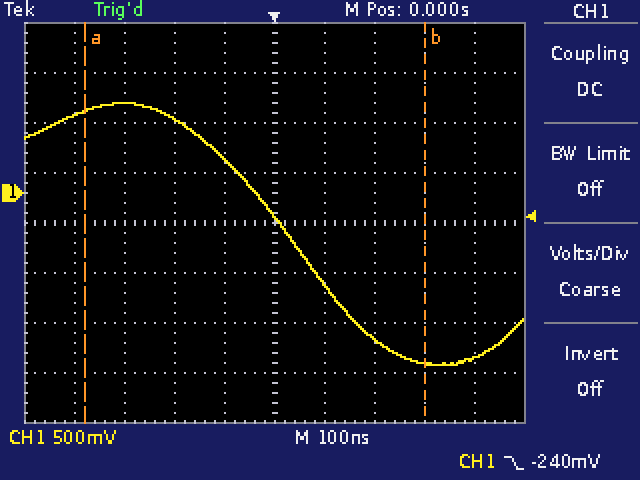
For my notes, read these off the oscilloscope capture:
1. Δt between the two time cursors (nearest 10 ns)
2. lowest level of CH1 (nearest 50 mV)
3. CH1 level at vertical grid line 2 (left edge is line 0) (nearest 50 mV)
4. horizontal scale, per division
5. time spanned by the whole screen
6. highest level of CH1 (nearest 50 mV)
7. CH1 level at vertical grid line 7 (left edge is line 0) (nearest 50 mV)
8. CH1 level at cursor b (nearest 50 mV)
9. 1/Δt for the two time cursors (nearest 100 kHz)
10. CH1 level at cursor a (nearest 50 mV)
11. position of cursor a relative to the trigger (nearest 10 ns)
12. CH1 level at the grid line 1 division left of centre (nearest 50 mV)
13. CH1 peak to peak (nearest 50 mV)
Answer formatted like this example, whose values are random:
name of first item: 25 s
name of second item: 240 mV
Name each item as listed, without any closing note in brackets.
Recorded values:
Δt between the two time cursors: 680 ns
lowest level of CH1: -1.70 V
CH1 level at vertical grid line 2 (left edge is line 0): 900 mV
horizontal scale, per division: 100 ns
time spanned by the whole screen: 1 µs
highest level of CH1: 900 mV
CH1 level at vertical grid line 7 (left edge is line 0): -1.45 V
CH1 level at cursor b: -1.70 V
1/Δt for the two time cursors: 1.5 MHz
CH1 level at cursor a: 800 mV
position of cursor a relative to the trigger: -380 ns
CH1 level at the grid line 1 division left of centre: 350 mV
CH1 peak to peak: 2.60 V
